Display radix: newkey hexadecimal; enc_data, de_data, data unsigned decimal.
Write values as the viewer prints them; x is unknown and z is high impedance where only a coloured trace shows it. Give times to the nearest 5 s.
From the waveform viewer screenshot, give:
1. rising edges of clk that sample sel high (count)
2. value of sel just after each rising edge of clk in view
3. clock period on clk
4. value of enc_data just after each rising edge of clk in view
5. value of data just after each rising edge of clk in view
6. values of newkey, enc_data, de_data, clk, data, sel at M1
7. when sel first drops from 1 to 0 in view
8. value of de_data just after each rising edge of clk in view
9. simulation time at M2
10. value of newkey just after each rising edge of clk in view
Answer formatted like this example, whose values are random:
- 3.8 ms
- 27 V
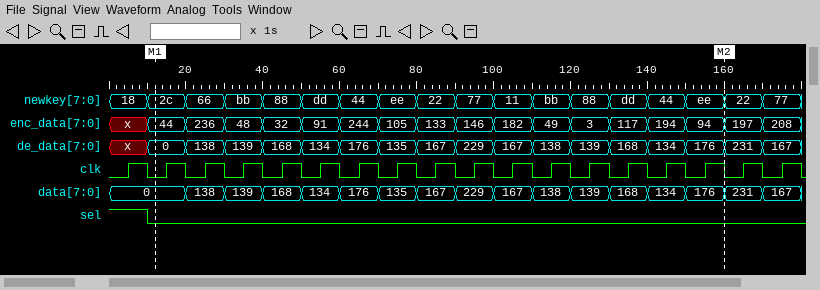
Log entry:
- 1
- 1 0 0 0 0 0 0 0 0 0 0 0 0 0 0 0 0 0
- 10 s
- x, 44, 236, 48, 32, 91, 244, 105, 133, 146, 182, 49, 3, 117, 194, 94, 197, 208
- 0, 0, 138, 139, 168, 134, 176, 135, 167, 229, 167, 138, 139, 168, 134, 176, 231, 167
- newkey=2c, enc_data=44, de_data=0, clk=0, data=0, sel=0
- 10 s
- x, 0, 138, 139, 168, 134, 176, 135, 167, 229, 167, 138, 139, 168, 134, 176, 231, 167
- 160 s
- 18, 2c, 66, bb, 88, dd, 44, ee, 22, 77, 11, bb, 88, dd, 44, ee, 22, 77
